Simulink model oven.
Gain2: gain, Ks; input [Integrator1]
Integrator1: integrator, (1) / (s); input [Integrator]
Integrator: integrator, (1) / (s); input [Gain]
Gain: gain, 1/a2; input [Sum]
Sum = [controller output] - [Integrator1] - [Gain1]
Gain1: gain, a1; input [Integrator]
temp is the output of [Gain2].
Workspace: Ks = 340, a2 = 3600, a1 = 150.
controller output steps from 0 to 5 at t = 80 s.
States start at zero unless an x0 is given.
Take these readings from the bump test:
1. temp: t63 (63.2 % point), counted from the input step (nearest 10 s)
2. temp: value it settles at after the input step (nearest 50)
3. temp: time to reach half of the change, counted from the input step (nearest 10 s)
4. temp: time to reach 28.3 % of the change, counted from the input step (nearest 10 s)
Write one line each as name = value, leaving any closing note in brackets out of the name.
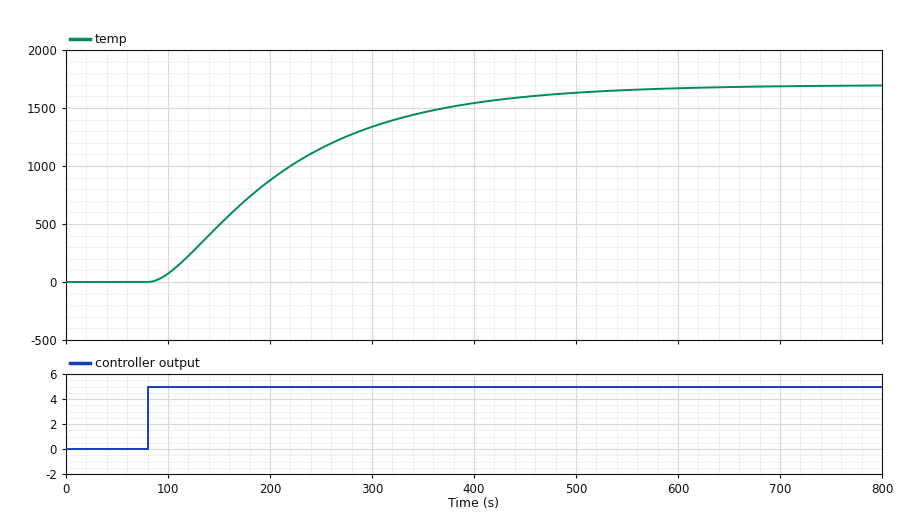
temp: t63 (63.2 % point), counted from the input step = 150 s
temp: value it settles at after the input step = 1700
temp: time to reach half of the change, counted from the input step = 120 s
temp: time to reach 28.3 % of the change, counted from the input step = 70 s
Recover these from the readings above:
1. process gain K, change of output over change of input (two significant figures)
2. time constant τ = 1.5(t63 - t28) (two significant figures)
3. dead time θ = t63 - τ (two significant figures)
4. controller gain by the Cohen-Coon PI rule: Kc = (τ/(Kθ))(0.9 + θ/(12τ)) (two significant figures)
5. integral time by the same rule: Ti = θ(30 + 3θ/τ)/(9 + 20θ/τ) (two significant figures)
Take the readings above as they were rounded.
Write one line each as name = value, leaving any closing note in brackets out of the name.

process gain K, change of output over change of input = 340
time constant τ = 1.5(t63 - t28) = 120 s
dead time θ = t63 - τ = 30 s
controller gain by the Cohen-Coon PI rule: Kc = (τ/(Kθ))(0.9 + θ/(12τ)) = 0.011
integral time by the same rule: Ti = θ(30 + 3θ/τ)/(9 + 20θ/τ) = 66 s
